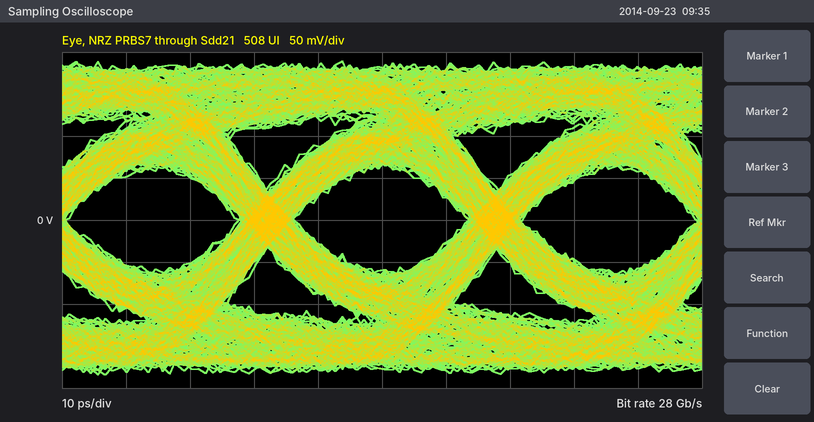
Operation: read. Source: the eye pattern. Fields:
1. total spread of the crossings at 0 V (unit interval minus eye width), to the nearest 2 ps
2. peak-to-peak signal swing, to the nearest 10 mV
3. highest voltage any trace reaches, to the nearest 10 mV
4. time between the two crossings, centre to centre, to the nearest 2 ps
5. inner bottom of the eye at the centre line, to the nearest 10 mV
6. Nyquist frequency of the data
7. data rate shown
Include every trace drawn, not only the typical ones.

8 ps
370 mV
190 mV
36 ps
-60 mV
14 GHz
28 Gb/s
